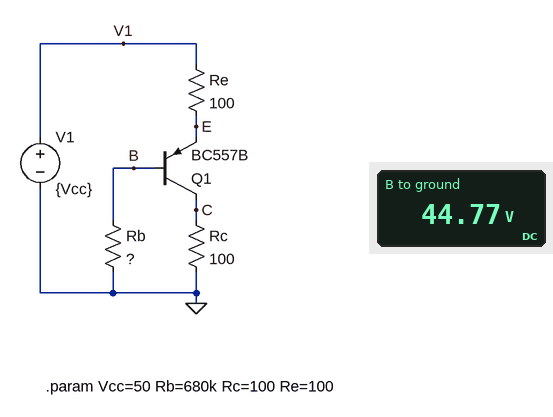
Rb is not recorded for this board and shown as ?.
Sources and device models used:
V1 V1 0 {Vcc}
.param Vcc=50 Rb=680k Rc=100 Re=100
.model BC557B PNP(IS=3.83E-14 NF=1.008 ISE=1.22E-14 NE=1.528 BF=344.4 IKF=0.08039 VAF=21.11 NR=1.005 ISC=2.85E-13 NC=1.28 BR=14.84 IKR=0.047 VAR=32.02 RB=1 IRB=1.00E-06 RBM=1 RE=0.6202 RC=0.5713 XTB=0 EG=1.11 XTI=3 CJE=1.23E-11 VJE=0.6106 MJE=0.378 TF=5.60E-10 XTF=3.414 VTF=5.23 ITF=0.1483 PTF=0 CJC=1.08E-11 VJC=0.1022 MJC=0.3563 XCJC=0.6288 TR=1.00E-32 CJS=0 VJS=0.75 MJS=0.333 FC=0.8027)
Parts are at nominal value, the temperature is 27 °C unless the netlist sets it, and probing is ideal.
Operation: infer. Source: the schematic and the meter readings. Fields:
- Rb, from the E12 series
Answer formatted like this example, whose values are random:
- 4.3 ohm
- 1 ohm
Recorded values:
- 820 kΩ
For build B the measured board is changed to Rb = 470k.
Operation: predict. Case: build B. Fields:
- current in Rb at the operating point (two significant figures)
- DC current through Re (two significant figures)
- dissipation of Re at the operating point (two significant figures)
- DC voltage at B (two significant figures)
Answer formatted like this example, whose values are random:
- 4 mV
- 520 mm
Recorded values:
- 91 µA
- 65 mA
- 420 mW
- 43 V
